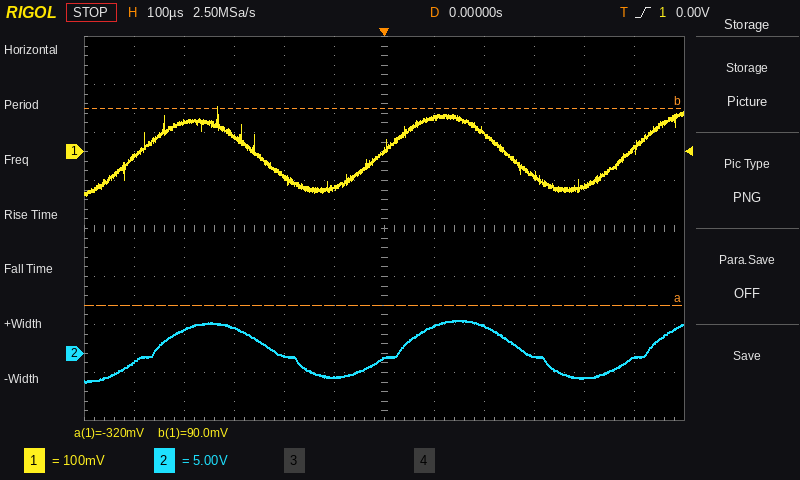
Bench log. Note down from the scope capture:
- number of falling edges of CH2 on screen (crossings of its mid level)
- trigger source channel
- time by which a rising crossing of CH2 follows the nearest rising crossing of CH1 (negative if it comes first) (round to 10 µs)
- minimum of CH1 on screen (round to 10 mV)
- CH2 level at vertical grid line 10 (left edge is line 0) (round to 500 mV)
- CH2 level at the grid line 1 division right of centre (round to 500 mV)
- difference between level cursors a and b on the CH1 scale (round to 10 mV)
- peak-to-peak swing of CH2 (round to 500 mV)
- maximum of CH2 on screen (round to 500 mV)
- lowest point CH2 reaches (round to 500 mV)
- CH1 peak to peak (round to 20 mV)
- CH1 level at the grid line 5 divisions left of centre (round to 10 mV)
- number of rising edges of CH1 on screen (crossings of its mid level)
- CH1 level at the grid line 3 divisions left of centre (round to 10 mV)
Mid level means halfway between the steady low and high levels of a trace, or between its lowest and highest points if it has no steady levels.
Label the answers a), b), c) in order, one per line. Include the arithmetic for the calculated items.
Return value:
a) 2
b) CH1
c) +30 µs
d) -90 mV
e) -2.5 V
f) 3.0 V
g) 410 mV
h) 3.5 V − (-3.0 V) = 6.5 V
i) 3.5 V
j) -3.0 V
k) 180 mV
l) -10 mV
m) 3
n) 30 mV
